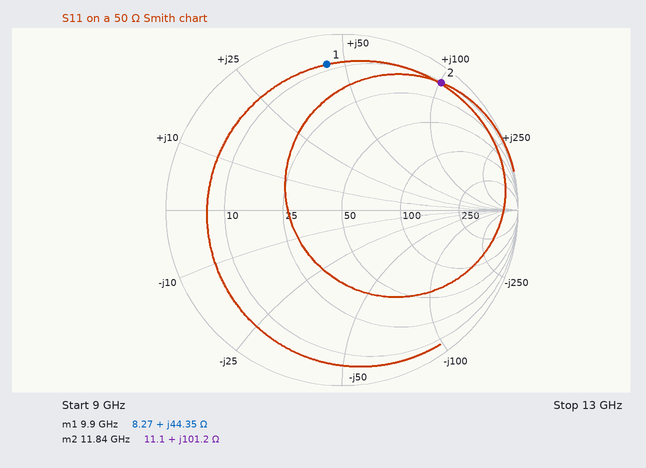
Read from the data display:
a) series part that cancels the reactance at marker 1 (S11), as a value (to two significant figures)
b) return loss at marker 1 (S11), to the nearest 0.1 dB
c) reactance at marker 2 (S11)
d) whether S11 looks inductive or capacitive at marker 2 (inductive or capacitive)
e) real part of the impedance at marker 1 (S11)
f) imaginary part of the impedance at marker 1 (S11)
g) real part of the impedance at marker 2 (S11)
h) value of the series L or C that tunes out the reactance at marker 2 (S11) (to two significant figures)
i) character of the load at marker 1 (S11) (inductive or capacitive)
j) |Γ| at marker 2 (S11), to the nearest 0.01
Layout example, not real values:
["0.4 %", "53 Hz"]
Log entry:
["360 fF", "1.6 dB", "+101.2 Ω", "inductive", "8.27 Ω", "+44.35 Ω", "11.1 Ω", "130 fF", "inductive", "0.92"]
